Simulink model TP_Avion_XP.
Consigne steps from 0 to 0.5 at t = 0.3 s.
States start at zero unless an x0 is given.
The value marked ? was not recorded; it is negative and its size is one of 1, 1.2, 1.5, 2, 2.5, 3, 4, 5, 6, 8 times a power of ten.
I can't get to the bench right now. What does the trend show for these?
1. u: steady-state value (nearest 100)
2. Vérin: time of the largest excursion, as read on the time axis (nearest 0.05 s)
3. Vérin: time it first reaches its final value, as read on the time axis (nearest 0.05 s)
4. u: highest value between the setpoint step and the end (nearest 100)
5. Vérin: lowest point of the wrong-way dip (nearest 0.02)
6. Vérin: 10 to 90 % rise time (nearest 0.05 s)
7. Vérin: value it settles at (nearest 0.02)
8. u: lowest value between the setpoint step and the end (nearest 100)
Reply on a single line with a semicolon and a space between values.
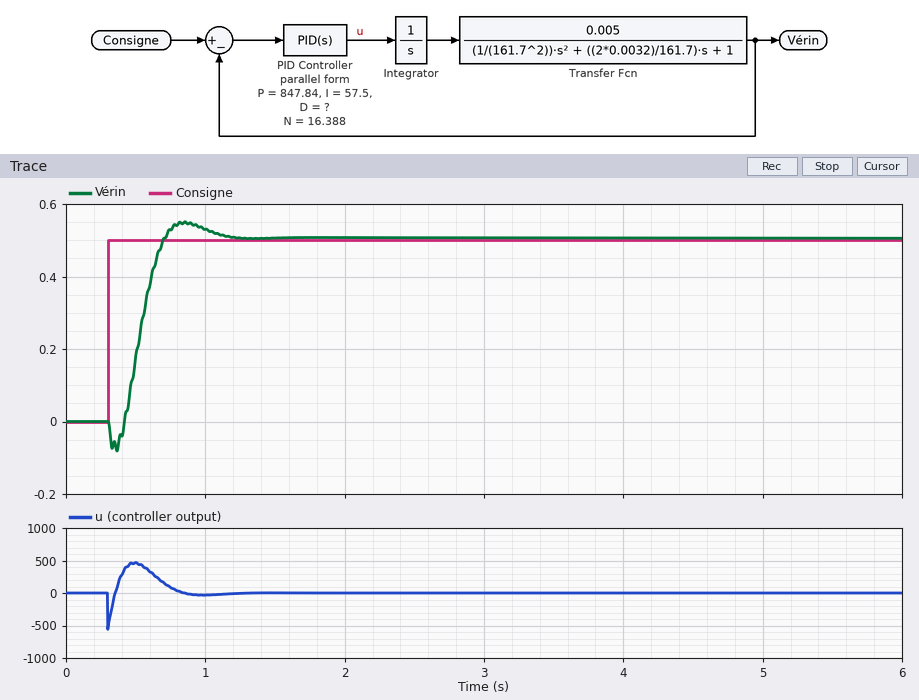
0; 0.85 s; 0.70 s; 500; -0.08; 0.20 s; 0.50; -600
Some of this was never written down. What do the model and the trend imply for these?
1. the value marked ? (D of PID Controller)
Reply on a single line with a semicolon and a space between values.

-120
